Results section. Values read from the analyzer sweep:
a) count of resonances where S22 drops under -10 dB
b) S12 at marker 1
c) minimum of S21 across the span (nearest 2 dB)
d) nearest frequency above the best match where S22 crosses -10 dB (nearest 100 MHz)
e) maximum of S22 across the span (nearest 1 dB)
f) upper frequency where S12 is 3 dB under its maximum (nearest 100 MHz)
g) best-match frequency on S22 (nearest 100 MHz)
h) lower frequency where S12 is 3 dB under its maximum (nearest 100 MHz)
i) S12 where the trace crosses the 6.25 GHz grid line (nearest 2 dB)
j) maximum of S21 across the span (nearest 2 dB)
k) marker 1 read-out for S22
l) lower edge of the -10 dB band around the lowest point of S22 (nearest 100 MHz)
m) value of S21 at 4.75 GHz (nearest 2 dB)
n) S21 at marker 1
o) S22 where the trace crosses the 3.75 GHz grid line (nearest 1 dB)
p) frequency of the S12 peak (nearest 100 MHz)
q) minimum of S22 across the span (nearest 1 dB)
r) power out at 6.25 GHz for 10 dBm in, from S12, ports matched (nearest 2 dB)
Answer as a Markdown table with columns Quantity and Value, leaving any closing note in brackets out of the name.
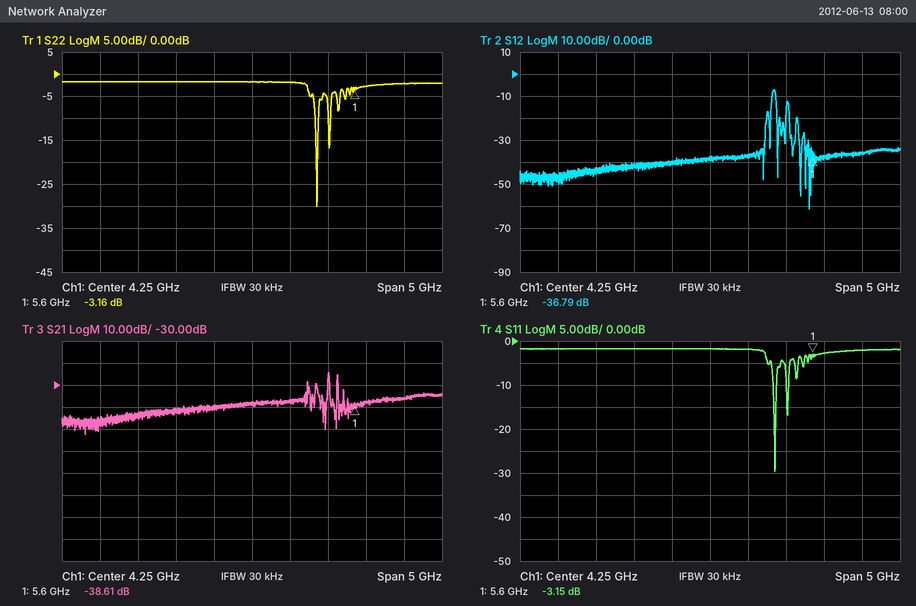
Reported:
| Quantity | Value |
|---|---|
| count of resonances where S22 drops under -10 dB | 2 |
| S12 at marker 1 | -36.79 dB |
| minimum of S21 across the span | -52 dB |
| nearest frequency above the best match where S22 crosses -10 dB | 5.1 GHz |
| maximum of S22 across the span | -2 dB |
| upper frequency where S12 is 3 dB under its maximum | 5.1 GHz |
| best-match frequency on S22 | 5.1 GHz |
| lower frequency where S12 is 3 dB under its maximum | 5.1 GHz |
| S12 where the trace crosses the 6.25 GHz grid line | -36 dB |
| maximum of S21 across the span | -24 dB |
| marker 1 read-out for S22 | -3.16 dB |
| lower edge of the -10 dB band around the lowest point of S22 | 5.1 GHz |
| value of S21 at 4.75 GHz | -38 dB |
| S21 at marker 1 | -38.61 dB |
| S22 where the trace crosses the 3.75 GHz grid line | -2 dB |
| frequency of the S12 peak | 5.1 GHz |
| minimum of S22 across the span | -30 dB |
| power out at 6.25 GHz for 10 dBm in, from S12, ports matched | -26 dBm |
